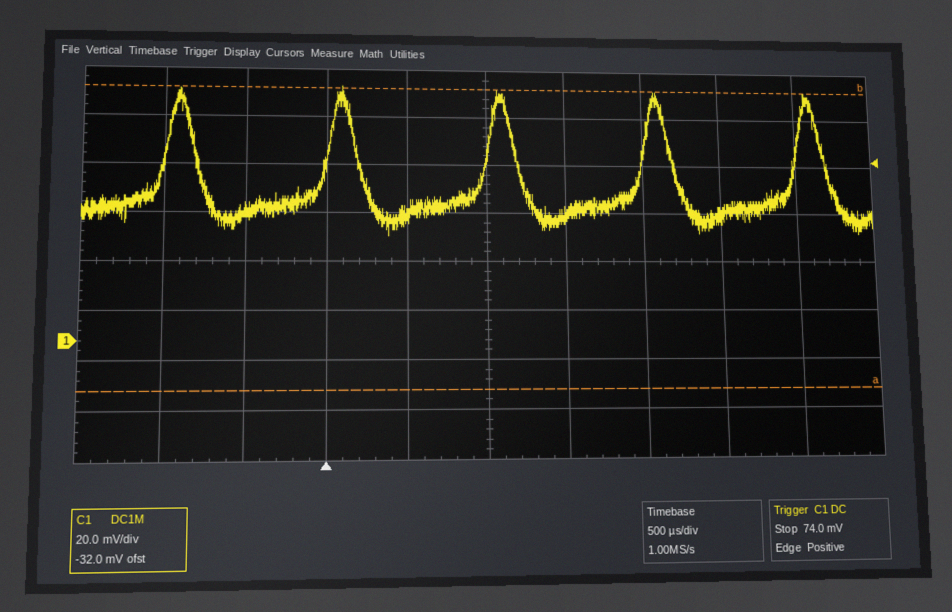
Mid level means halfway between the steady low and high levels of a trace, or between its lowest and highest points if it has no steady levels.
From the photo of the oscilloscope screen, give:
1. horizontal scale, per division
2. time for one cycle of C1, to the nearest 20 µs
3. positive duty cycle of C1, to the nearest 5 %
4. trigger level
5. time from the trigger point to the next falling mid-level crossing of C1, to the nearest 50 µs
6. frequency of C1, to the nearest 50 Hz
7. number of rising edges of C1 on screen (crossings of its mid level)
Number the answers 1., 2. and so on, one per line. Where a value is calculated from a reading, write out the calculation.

1. 500 µs
2. 1.00 ms
3. 20 %
4. 74.0 mV
5. 200 µs
6. 1 / 1.00 ms ≈ 1.00 kHz
7. 5
